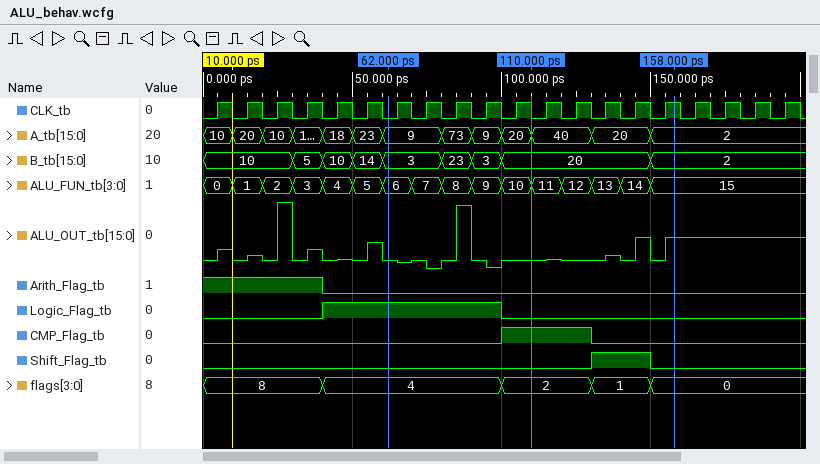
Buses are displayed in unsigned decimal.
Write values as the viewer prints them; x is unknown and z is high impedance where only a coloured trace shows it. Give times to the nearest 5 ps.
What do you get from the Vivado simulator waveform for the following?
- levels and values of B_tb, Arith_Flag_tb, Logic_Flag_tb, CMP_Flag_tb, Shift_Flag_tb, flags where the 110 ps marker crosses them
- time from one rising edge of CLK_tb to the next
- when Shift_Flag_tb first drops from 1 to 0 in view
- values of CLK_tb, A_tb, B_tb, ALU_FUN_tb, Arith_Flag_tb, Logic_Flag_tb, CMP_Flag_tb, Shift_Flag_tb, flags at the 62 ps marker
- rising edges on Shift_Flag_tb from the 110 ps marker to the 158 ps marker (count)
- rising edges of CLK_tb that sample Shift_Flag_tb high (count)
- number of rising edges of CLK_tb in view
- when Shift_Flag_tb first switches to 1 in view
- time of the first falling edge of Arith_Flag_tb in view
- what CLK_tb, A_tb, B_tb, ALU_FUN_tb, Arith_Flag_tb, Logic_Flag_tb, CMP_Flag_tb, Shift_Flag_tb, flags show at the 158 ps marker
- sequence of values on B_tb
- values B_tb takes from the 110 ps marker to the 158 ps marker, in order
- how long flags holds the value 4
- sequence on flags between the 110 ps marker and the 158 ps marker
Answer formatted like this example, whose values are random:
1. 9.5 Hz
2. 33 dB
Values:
1. B_tb=20, Arith_Flag_tb=0, Logic_Flag_tb=0, CMP_Flag_tb=1, Shift_Flag_tb=0, flags=2
2. 10 ps
3. 150 ps
4. CLK_tb=0, A_tb=9, B_tb=3, ALU_FUN_tb=6, Arith_Flag_tb=0, Logic_Flag_tb=1, CMP_Flag_tb=0, Shift_Flag_tb=0, flags=4
5. 1
6. 2
7. 20
8. 130 ps
9. 40 ps
10. CLK_tb=1, A_tb=2, B_tb=2, ALU_FUN_tb=15, Arith_Flag_tb=0, Logic_Flag_tb=0, CMP_Flag_tb=0, Shift_Flag_tb=0, flags=0
11. 10, 5, 10, 14, 3, 23, 3, 20, 2
12. 20, 2
13. 60 ps
14. 2, 1, 0
